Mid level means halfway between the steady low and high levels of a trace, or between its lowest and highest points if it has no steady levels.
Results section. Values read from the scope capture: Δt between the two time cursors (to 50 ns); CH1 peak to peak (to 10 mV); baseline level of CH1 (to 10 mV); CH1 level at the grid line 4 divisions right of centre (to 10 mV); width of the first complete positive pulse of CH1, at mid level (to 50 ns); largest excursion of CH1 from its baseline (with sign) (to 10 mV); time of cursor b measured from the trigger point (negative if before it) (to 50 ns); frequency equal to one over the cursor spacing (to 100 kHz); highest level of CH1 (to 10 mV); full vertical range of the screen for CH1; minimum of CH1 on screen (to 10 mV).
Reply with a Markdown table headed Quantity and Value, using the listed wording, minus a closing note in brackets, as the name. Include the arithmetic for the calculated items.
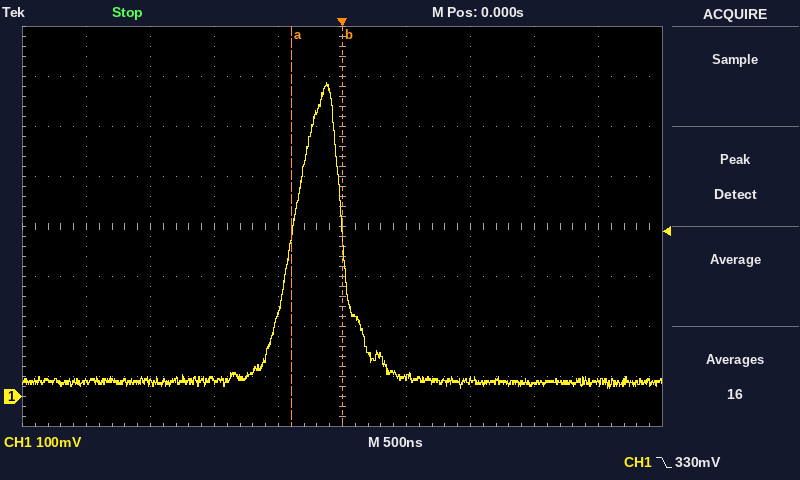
| Quantity | Value |
|---|---|
| Δt between the two time cursors | 400 ns |
| CH1 peak to peak | 630 mV − (20 mV) = 610 mV |
| baseline level of CH1 | 30 mV |
| CH1 level at the grid line 4 divisions right of centre | 30 mV |
| width of the first complete positive pulse of CH1, at mid level | 400 ns |
| largest excursion of CH1 from its baseline (with sign) | 630 mV − (30 mV) = +600 mV |
| time of cursor b measured from the trigger point (negative if before it) | 0 ns |
| frequency equal to one over the cursor spacing | 1 / 400 ns ≈ 2.5 MHz |
| highest level of CH1 | 630 mV |
| full vertical range of the screen for CH1 | 800 mV |
| minimum of CH1 on screen | 20 mV |
